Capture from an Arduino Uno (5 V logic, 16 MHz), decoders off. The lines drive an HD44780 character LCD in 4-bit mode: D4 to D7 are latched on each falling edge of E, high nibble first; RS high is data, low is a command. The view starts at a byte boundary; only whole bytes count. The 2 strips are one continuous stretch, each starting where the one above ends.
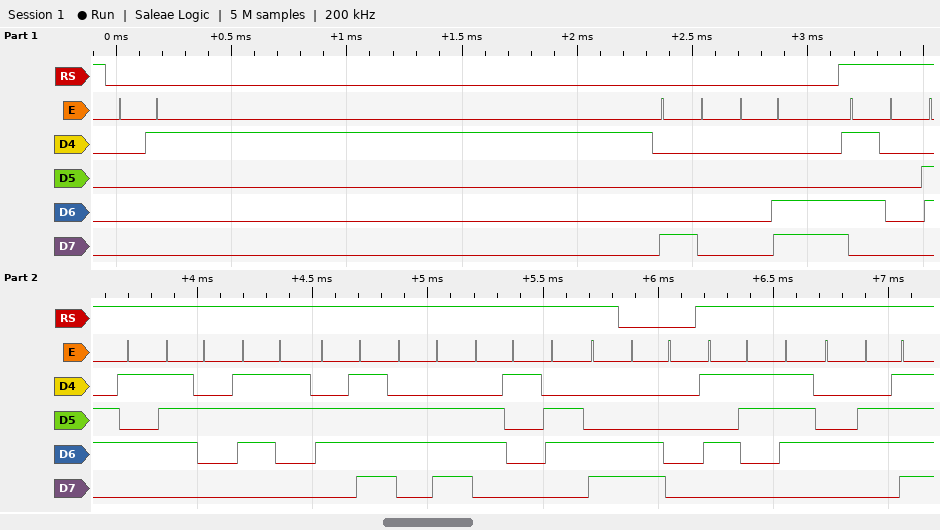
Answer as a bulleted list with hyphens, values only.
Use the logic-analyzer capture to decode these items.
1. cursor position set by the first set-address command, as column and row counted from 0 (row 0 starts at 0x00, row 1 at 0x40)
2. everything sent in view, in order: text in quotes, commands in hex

- column 0, row 0
- 0x01 0x80 0x0C "Personal" 0xC0 "Sto"
